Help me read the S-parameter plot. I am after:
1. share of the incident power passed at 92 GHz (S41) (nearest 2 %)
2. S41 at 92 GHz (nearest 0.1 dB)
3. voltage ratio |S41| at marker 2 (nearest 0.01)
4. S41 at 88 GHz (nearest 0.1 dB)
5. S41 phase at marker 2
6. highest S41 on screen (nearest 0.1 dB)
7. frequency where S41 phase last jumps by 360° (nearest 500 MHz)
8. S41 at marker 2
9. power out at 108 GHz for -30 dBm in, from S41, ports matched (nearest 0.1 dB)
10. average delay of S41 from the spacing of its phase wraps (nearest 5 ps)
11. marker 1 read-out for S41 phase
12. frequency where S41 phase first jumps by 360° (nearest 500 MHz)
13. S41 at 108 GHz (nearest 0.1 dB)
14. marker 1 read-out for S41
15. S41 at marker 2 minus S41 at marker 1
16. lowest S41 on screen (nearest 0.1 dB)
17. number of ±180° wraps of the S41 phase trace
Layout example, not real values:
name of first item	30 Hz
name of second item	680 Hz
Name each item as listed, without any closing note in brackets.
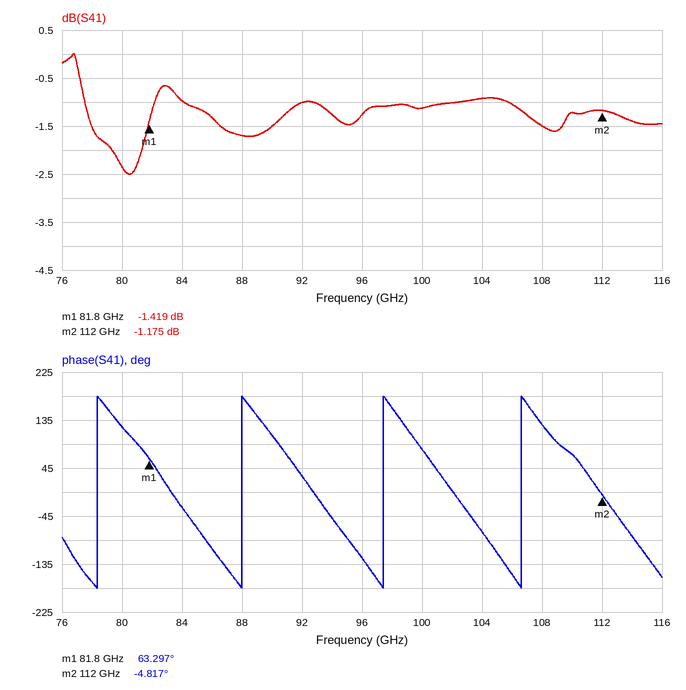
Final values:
share of the incident power passed at 92 GHz (S41)	80 %
S41 at 92 GHz	-1.0 dB
voltage ratio |S41| at marker 2	0.87
S41 at 88 GHz	-1.7 dB
S41 phase at marker 2	-4.817°
highest S41 on screen	0.0 dB
frequency where S41 phase last jumps by 360°	106.5 GHz
S41 at marker 2	-1.175 dB
power out at 108 GHz for -30 dBm in, from S41, ports matched	-31.5 dBm
average delay of S41 from the spacing of its phase wraps	105 ps
marker 1 read-out for S41 phase	63.297°
frequency where S41 phase first jumps by 360°	78.5 GHz
S41 at 108 GHz	-1.5 dB
marker 1 read-out for S41	-1.419 dB
S41 at marker 2 minus S41 at marker 1	0.244 dB
lowest S41 on screen	-2.5 dB
number of ±180° wraps of the S41 phase trace	4
